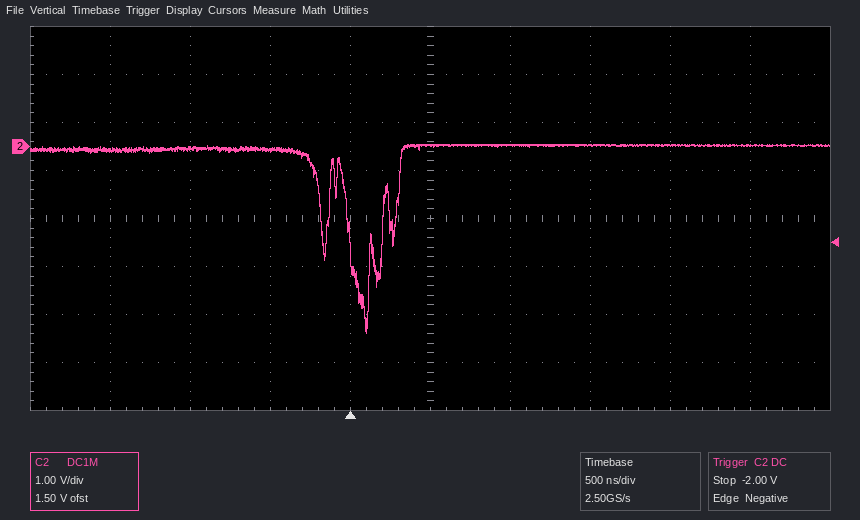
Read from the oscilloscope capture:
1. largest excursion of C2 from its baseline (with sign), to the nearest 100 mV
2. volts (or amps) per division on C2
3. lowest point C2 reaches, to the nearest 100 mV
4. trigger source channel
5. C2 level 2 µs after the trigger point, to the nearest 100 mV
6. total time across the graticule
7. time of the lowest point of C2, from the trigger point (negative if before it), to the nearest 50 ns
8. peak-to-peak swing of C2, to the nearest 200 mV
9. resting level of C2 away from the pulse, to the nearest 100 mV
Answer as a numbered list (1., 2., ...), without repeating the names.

1. -3.9 V
2. 1 V
3. -3.9 V
4. C2
5. 0.0 V
6. 5 µs
7. +100 ns
8. 4.0 V
9. 0.0 V
